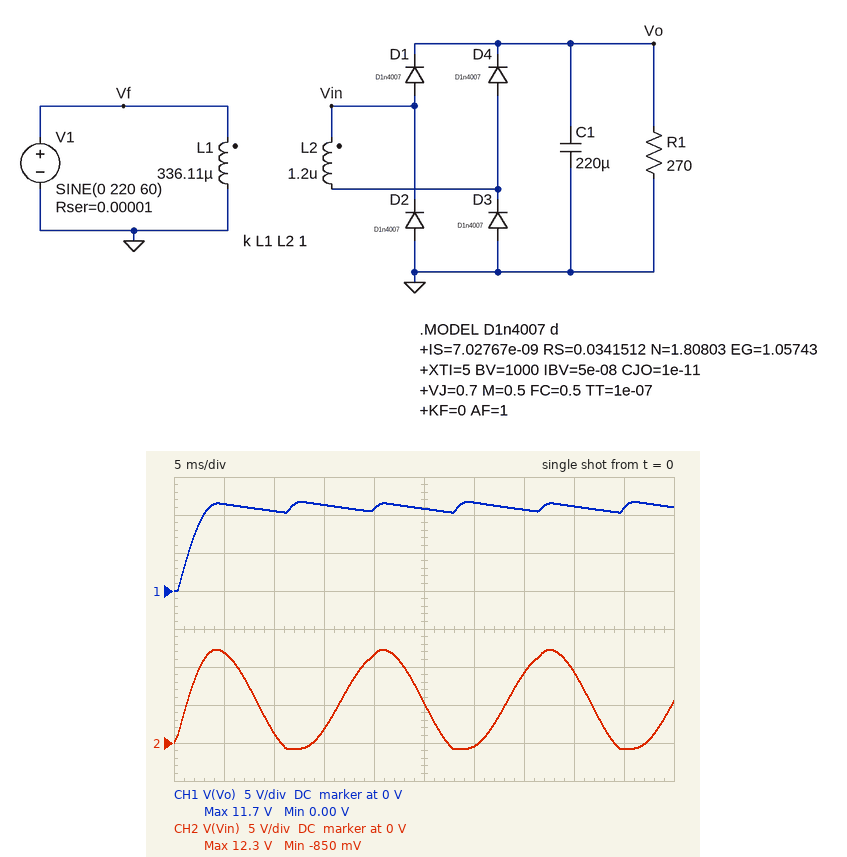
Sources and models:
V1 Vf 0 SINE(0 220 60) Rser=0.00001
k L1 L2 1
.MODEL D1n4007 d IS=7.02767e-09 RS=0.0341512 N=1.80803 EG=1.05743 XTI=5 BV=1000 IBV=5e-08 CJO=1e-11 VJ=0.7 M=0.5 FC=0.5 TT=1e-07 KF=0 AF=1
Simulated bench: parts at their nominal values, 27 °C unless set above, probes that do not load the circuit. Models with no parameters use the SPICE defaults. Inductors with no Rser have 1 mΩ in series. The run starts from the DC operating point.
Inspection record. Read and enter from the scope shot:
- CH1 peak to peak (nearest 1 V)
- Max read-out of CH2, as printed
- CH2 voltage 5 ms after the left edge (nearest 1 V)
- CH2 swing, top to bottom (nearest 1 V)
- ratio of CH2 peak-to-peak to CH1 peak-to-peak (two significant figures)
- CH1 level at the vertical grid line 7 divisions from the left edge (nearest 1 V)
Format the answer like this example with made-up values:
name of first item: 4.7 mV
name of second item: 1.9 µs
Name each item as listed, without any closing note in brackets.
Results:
CH1 peak to peak: 12 V
Max read-out of CH2, as printed: 12.3 V
CH2 voltage 5 ms after the left edge: 12 V
CH2 swing, top to bottom: 13 V
ratio of CH2 peak-to-peak to CH1 peak-to-peak: 1.1
CH1 level at the vertical grid line 7 divisions from the left edge: 11 V
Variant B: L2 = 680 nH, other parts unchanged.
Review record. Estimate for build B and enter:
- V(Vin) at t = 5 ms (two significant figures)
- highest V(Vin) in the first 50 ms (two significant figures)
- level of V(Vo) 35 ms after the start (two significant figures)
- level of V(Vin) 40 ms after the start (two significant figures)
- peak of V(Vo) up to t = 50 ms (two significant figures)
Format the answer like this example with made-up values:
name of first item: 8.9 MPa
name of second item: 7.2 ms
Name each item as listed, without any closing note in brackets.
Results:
V(Vin) at t = 5 ms: 8.8 V
highest V(Vin) in the first 50 ms: 9.1 V
level of V(Vo) 35 ms after the start: 7.7 V
level of V(Vin) 40 ms after the start: 6.9 V
peak of V(Vo) up to t = 50 ms: 8.5 V
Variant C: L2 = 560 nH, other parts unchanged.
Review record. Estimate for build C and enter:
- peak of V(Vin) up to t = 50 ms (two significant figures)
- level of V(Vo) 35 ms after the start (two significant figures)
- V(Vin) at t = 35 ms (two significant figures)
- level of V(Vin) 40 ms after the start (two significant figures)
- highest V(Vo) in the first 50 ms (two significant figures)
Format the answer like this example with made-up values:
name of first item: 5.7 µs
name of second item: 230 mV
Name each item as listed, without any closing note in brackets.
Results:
peak of V(Vin) up to t = 50 ms: 8.2 V
level of V(Vo) 35 ms after the start: 6.9 V
V(Vin) at t = 35 ms: 6.1 V
level of V(Vin) 40 ms after the start: 6.2 V
highest V(Vo) in the first 50 ms: 7.6 V
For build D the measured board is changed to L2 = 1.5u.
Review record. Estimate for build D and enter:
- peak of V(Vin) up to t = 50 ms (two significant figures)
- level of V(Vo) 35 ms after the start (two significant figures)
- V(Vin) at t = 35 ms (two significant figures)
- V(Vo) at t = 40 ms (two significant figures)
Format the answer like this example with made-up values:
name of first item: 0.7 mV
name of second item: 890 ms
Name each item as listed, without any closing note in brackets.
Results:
peak of V(Vin) up to t = 50 ms: 14 V
level of V(Vo) 35 ms after the start: 12 V
V(Vin) at t = 35 ms: 10 V
V(Vo) at t = 40 ms: 13 V
